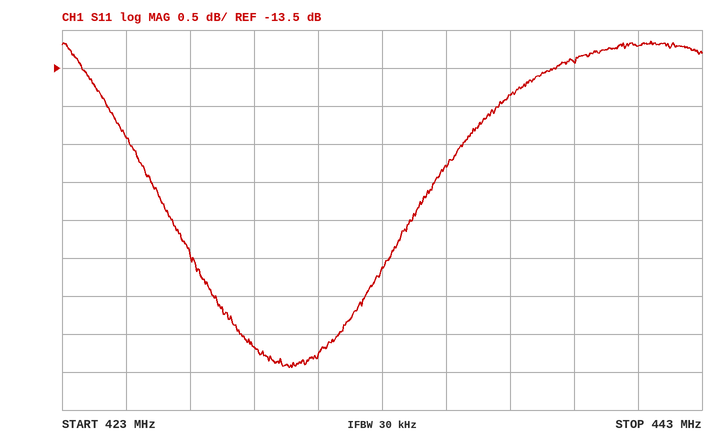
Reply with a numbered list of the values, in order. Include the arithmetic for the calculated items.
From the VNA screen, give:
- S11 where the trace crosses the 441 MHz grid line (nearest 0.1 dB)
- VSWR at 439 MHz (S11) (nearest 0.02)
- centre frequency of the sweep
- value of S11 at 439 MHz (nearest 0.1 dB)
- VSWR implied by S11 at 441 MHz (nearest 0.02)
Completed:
1. -13.2 dB
2. |Γ| = 10^(-13.4/20) = 0.2138; VSWR = (1 + 0.2138)/(1 − 0.2138) ≈ 1.54
3. 433 MHz
4. -13.4 dB
5. |Γ| = 10^(-13.2/20) = 0.2188; VSWR = (1 + 0.2188)/(1 − 0.2188) ≈ 1.56
